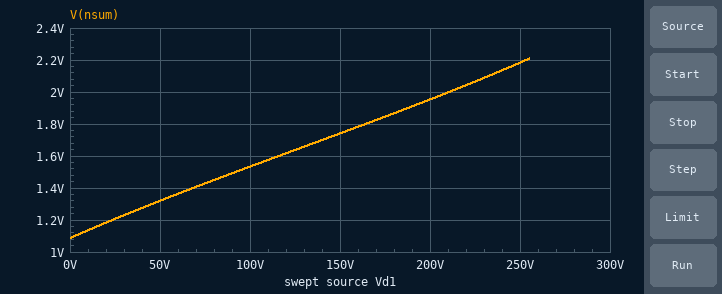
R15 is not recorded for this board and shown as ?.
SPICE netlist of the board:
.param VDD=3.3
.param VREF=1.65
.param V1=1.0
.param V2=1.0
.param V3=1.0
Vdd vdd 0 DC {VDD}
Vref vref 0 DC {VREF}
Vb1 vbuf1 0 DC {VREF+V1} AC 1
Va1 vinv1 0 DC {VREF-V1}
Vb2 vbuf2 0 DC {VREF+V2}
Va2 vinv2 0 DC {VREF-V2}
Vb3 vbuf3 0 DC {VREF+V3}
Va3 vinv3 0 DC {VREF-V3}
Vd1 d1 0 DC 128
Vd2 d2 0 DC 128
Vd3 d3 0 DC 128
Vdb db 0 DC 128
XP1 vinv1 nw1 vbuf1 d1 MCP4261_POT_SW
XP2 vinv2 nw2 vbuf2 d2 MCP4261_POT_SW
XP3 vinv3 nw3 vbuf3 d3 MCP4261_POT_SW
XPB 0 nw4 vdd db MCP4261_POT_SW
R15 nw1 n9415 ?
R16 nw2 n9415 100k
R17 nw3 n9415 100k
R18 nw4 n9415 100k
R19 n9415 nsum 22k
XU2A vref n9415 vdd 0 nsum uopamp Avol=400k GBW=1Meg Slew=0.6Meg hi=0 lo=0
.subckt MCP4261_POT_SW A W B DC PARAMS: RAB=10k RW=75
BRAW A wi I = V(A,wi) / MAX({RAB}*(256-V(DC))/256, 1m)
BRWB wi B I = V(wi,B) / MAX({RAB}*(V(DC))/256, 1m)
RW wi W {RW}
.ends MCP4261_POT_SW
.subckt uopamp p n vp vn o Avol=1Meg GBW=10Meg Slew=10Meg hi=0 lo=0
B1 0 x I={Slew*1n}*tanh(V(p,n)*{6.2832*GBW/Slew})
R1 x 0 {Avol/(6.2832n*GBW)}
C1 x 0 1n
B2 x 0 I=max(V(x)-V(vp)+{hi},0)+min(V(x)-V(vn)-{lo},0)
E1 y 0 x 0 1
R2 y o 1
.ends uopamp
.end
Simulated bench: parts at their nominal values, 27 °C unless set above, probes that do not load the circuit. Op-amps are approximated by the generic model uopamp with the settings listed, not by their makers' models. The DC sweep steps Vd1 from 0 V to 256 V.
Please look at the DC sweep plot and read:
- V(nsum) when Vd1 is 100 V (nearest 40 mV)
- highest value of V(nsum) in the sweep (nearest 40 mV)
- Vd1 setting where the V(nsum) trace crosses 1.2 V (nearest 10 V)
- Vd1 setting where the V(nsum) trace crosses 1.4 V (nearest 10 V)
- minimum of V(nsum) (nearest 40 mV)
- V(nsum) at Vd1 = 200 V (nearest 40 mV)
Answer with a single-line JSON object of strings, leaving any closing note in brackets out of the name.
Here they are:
{"V(nsum) when Vd1 is 100 V": "1.52 V", "highest value of V(nsum) in the sweep": "2.20 V", "Vd1 setting where the V(nsum) trace crosses 1.2 V": "20 V", "Vd1 setting where the V(nsum) trace crosses 1.4 V": "70 V", "minimum of V(nsum)": "1.08 V", "V(nsum) at Vd1 = 200 V": "1.96 V"}
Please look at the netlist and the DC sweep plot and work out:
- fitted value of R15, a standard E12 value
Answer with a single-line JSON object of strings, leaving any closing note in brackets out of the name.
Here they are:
{"fitted value of R15, a standard E12 value": "39 kΩ"}
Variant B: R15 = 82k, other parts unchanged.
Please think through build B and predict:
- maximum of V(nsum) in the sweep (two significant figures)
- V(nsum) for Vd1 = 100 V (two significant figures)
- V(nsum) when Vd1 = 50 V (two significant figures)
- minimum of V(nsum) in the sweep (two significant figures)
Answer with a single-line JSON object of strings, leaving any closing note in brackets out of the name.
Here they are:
{"maximum of V(nsum) in the sweep": "1.9 V", "V(nsum) for Vd1 = 100 V": "1.6 V", "V(nsum) when Vd1 = 50 V": "1.5 V", "minimum of V(nsum) in the sweep": "1.4 V"}
